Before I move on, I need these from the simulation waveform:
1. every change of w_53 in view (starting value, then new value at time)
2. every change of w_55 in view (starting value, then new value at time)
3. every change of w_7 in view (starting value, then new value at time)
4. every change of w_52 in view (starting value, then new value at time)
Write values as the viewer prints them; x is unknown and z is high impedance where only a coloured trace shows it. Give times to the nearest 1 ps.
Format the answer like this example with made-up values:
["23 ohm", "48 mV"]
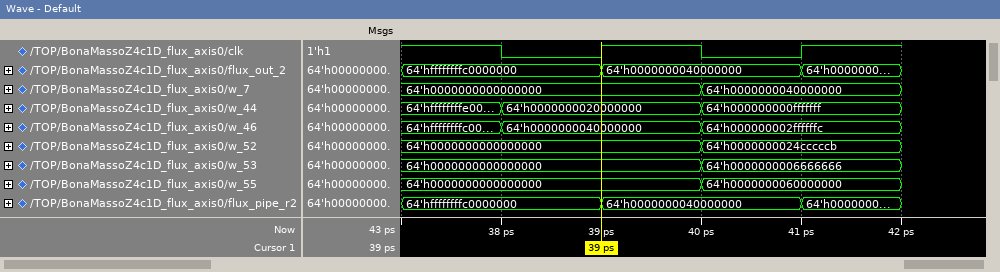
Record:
["64'h0000000000000000, 64'h0000000006666666 at 40 ps", "64'h0000000000000000, 64'h0000000060000000 at 40 ps", "64'h0000000000000000, 64'h0000000040000000 at 40 ps", "64'h0000000000000000, 64'h0000000024cccccb at 40 ps"]
